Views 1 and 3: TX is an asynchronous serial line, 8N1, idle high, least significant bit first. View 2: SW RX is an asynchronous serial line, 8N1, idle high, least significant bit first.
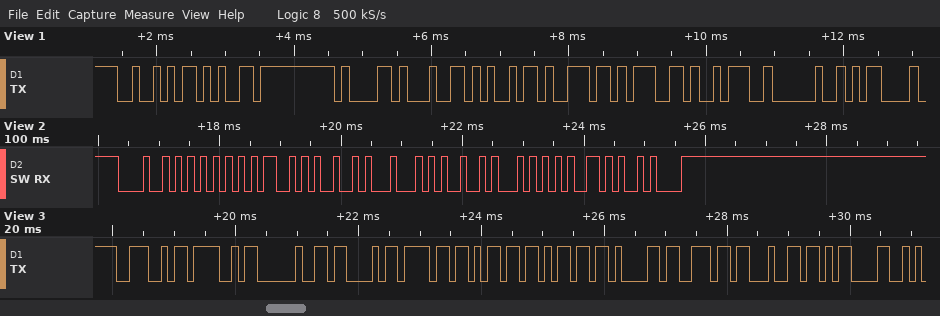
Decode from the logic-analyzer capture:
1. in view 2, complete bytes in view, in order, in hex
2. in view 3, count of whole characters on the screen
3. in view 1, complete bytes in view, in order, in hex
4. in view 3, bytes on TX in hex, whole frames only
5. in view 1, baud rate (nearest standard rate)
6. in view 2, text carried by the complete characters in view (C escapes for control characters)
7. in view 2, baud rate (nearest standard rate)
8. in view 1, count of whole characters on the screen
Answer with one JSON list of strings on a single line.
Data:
["48 55 4D 49 44 49 54 59 0A", "11", "52 65 61 64 69 6E 67 3A 20 0D", "4E 4F 20 43 6F 6D 6D 61 6E 64 0D", "9600 baud", "\"HUMIDITY\\n\"", "9600 baud", "10"]
